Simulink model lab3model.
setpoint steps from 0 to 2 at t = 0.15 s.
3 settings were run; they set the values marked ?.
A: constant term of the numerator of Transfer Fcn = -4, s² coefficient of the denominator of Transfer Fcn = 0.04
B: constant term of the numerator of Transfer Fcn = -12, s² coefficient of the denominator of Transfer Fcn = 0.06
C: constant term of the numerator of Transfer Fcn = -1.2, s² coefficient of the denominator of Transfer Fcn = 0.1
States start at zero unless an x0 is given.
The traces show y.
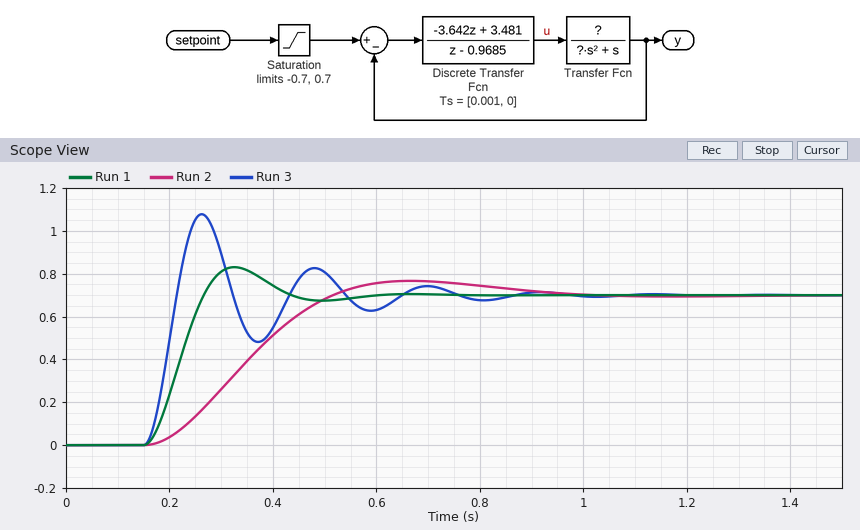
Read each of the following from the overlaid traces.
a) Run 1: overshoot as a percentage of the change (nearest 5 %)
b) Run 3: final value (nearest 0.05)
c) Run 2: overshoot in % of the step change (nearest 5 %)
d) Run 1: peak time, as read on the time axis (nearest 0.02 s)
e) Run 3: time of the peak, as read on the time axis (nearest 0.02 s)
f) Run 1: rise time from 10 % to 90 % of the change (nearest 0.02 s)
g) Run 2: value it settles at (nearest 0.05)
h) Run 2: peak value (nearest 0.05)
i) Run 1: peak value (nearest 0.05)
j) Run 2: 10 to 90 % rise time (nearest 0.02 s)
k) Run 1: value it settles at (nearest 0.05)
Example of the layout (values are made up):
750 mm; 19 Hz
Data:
20 %; 0.70; 10 %; 0.32 s; 0.26 s; 0.08 s; 0.70; 0.75; 0.85; 0.24 s; 0.70
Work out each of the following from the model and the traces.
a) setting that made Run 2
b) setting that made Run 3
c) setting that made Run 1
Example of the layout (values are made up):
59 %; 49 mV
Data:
C; B; A
